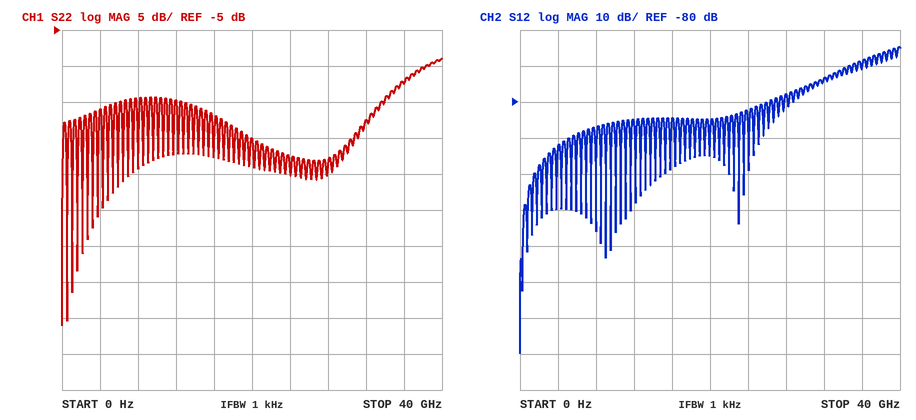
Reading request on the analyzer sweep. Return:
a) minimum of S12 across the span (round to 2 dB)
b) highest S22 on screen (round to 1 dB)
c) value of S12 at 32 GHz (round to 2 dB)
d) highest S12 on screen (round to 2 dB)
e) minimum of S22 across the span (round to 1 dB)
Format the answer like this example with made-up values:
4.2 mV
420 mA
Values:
-150 dB
-9 dB
-74 dB
-64 dB
-46 dB
